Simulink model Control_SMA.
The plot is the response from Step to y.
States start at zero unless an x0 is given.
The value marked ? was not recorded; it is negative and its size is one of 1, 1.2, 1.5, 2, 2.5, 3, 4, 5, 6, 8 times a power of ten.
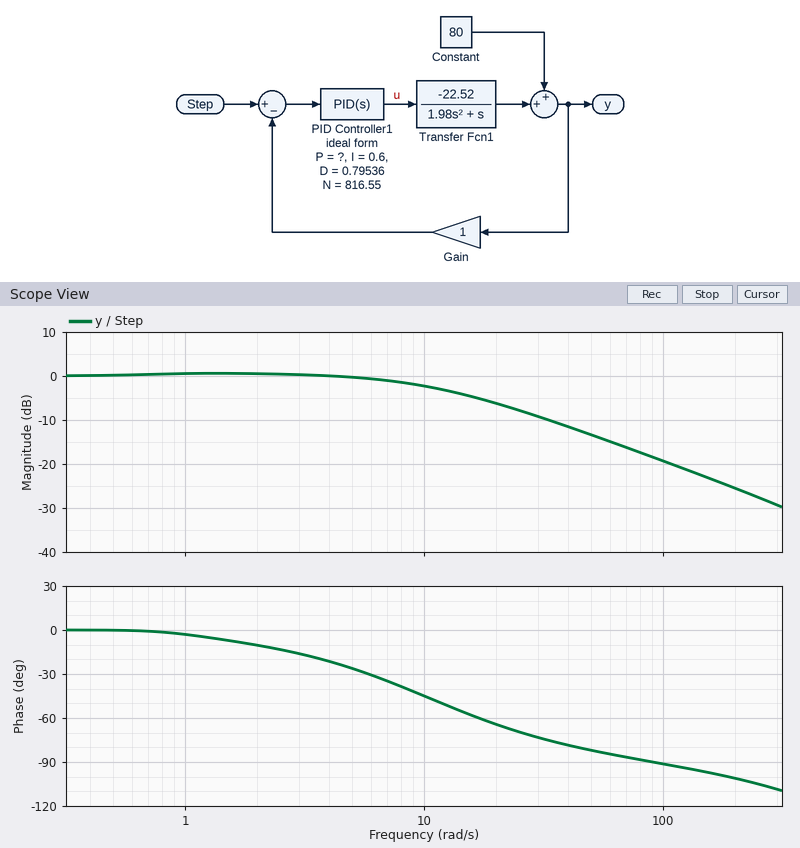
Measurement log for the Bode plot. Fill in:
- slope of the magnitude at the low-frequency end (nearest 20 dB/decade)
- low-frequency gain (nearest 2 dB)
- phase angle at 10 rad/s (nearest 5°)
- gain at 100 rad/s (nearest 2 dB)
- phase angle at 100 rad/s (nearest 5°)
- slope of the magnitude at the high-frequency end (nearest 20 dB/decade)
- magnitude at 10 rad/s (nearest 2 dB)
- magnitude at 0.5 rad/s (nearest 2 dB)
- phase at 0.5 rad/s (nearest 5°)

0 dB/decade
0 dB
-45°
-20 dB
-90°
-20 dB/decade
-2 dB
0 dB
0°
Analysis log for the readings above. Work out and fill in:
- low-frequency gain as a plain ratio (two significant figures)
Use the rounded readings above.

1.0
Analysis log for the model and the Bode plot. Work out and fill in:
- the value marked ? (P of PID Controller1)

-1.2
